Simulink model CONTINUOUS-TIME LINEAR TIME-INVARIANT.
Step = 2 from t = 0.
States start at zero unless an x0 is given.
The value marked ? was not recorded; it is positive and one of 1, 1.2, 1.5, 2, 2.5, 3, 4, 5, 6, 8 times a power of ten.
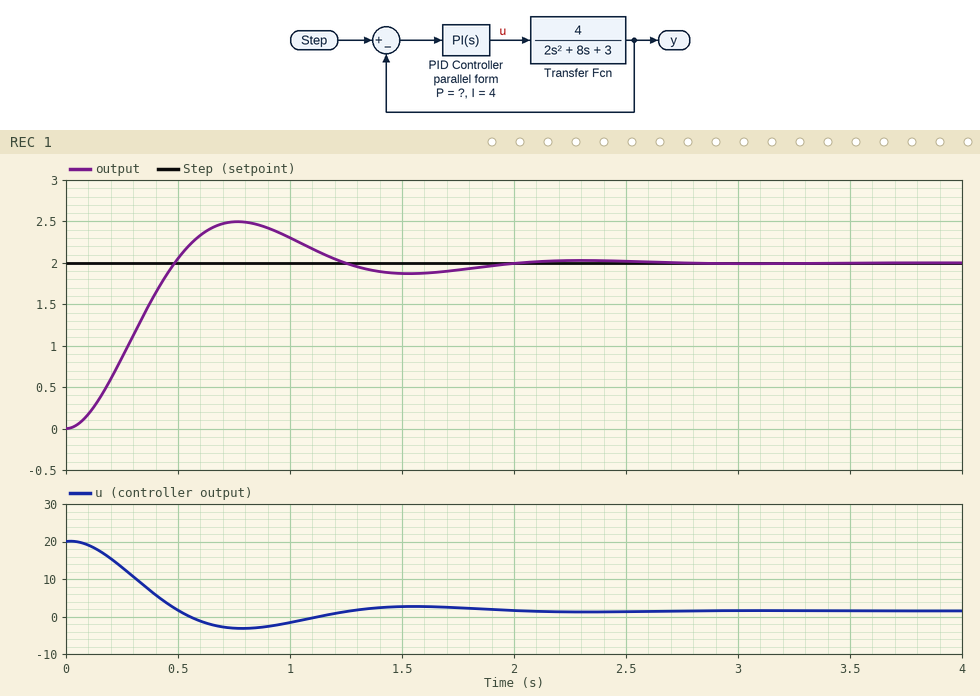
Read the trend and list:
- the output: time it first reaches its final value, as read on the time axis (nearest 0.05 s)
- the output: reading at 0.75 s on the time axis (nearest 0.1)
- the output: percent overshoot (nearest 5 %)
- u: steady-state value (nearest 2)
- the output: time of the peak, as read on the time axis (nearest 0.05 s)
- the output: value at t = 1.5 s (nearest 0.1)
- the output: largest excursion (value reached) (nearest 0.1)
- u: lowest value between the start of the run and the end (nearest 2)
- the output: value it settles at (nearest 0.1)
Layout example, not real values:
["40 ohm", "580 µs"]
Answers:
["0.50 s", "2.5", "25 %", "2", "0.75 s", "1.9", "2.5", "-4", "2.0"]
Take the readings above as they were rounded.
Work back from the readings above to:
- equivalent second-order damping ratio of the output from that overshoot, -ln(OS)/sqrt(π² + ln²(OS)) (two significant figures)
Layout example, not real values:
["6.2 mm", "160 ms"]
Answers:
["0.40"]
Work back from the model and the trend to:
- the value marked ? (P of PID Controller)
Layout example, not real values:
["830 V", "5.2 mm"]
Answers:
["10"]
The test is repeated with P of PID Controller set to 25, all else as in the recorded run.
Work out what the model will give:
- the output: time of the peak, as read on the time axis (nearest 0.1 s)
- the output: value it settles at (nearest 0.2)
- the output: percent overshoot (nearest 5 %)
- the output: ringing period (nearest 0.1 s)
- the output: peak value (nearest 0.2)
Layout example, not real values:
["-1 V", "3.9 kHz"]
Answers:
["0.5 s", "2.0", "40 %", "0.9 s", "2.8"]
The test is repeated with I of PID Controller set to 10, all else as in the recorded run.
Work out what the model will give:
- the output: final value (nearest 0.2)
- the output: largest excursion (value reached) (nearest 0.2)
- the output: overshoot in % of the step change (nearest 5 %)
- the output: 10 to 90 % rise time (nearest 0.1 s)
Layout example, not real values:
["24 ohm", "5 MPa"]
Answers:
["2.0", "2.8", "40 %", "0.3 s"]
